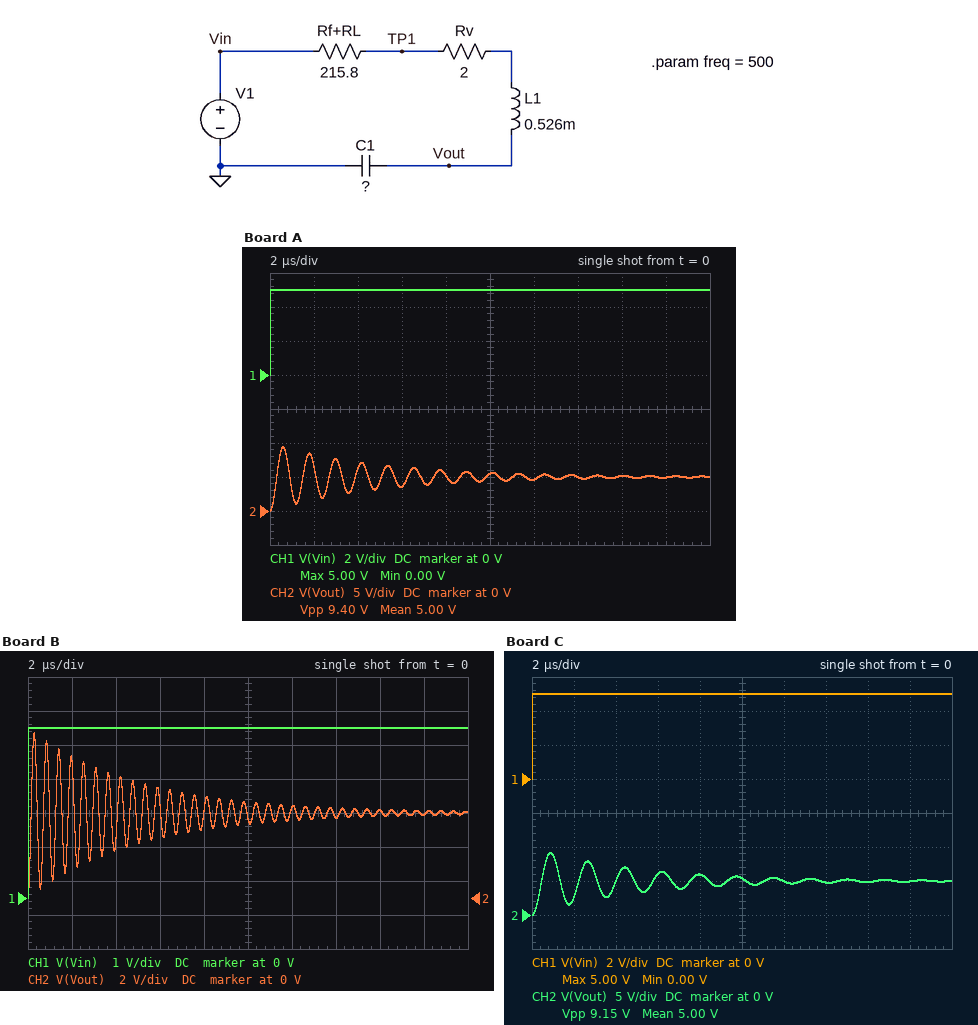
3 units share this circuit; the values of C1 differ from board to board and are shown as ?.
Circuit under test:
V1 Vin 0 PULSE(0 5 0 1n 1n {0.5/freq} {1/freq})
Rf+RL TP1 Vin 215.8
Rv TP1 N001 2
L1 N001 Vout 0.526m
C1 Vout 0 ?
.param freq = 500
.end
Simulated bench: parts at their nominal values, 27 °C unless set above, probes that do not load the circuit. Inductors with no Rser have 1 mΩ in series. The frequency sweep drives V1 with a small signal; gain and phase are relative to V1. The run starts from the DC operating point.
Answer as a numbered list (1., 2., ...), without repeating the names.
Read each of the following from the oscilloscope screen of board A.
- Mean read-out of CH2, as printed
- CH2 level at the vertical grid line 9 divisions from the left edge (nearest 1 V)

1. 5.00 V
2. 5 V
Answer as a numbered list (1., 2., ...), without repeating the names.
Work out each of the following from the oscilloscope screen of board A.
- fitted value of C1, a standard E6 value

1. 68 pF
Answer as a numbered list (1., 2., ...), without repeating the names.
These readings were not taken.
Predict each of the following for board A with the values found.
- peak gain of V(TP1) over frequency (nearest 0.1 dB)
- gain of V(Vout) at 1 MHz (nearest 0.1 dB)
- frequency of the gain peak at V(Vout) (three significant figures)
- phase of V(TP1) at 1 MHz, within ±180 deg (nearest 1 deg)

1. 0 dB
2. 7.5 dB
3. 840 kHz
4. 13 deg
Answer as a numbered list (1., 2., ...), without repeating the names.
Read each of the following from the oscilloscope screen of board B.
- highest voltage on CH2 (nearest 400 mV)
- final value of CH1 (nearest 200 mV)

1. 9.6 V
2. 5.0 V
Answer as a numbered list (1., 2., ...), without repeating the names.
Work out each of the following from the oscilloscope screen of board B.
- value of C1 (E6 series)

1. 15 pF
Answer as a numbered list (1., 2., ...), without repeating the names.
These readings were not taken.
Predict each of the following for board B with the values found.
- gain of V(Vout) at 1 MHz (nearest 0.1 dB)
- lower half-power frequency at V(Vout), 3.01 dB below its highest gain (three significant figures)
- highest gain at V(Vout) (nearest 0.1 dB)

1. 3.2 dB
2. 1.76 MHz
3. 28.7 dB
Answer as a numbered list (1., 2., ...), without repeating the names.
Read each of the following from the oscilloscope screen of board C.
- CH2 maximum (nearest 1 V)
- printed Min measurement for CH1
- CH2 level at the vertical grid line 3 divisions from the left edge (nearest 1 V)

1. 9 V
2. 0.00 V
3. 6 V
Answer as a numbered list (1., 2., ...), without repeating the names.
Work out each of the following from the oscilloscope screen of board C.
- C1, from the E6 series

1. 150 pF
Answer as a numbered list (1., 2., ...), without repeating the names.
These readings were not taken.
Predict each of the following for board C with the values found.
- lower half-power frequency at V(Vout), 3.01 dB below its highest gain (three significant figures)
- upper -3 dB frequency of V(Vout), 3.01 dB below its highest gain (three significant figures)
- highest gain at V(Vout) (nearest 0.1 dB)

1. 531 kHz
2. 597 kHz
3. 18.7 dB
